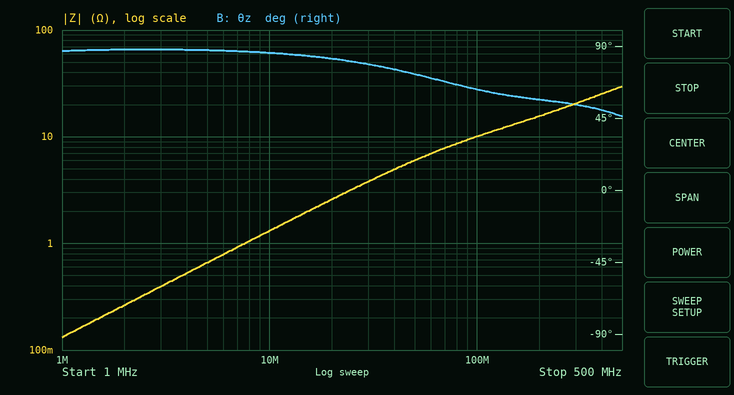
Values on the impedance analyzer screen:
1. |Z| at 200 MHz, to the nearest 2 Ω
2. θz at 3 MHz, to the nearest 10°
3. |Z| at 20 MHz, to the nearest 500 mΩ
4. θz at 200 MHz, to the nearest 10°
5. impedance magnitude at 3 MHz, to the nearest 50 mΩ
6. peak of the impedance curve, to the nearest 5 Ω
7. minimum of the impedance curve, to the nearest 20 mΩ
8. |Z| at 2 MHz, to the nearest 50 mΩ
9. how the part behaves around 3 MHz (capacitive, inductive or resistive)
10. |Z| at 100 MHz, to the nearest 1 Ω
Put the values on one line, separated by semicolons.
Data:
16 Ω; 90°; 2.5 Ω; 60°; 400 mΩ; 30 Ω; 140 mΩ; 250 mΩ; inductive; 10 Ω
